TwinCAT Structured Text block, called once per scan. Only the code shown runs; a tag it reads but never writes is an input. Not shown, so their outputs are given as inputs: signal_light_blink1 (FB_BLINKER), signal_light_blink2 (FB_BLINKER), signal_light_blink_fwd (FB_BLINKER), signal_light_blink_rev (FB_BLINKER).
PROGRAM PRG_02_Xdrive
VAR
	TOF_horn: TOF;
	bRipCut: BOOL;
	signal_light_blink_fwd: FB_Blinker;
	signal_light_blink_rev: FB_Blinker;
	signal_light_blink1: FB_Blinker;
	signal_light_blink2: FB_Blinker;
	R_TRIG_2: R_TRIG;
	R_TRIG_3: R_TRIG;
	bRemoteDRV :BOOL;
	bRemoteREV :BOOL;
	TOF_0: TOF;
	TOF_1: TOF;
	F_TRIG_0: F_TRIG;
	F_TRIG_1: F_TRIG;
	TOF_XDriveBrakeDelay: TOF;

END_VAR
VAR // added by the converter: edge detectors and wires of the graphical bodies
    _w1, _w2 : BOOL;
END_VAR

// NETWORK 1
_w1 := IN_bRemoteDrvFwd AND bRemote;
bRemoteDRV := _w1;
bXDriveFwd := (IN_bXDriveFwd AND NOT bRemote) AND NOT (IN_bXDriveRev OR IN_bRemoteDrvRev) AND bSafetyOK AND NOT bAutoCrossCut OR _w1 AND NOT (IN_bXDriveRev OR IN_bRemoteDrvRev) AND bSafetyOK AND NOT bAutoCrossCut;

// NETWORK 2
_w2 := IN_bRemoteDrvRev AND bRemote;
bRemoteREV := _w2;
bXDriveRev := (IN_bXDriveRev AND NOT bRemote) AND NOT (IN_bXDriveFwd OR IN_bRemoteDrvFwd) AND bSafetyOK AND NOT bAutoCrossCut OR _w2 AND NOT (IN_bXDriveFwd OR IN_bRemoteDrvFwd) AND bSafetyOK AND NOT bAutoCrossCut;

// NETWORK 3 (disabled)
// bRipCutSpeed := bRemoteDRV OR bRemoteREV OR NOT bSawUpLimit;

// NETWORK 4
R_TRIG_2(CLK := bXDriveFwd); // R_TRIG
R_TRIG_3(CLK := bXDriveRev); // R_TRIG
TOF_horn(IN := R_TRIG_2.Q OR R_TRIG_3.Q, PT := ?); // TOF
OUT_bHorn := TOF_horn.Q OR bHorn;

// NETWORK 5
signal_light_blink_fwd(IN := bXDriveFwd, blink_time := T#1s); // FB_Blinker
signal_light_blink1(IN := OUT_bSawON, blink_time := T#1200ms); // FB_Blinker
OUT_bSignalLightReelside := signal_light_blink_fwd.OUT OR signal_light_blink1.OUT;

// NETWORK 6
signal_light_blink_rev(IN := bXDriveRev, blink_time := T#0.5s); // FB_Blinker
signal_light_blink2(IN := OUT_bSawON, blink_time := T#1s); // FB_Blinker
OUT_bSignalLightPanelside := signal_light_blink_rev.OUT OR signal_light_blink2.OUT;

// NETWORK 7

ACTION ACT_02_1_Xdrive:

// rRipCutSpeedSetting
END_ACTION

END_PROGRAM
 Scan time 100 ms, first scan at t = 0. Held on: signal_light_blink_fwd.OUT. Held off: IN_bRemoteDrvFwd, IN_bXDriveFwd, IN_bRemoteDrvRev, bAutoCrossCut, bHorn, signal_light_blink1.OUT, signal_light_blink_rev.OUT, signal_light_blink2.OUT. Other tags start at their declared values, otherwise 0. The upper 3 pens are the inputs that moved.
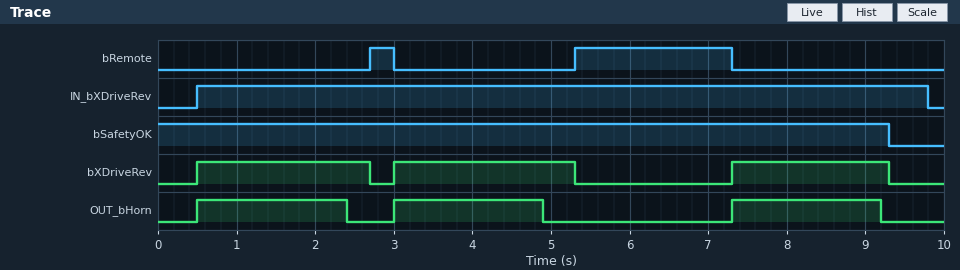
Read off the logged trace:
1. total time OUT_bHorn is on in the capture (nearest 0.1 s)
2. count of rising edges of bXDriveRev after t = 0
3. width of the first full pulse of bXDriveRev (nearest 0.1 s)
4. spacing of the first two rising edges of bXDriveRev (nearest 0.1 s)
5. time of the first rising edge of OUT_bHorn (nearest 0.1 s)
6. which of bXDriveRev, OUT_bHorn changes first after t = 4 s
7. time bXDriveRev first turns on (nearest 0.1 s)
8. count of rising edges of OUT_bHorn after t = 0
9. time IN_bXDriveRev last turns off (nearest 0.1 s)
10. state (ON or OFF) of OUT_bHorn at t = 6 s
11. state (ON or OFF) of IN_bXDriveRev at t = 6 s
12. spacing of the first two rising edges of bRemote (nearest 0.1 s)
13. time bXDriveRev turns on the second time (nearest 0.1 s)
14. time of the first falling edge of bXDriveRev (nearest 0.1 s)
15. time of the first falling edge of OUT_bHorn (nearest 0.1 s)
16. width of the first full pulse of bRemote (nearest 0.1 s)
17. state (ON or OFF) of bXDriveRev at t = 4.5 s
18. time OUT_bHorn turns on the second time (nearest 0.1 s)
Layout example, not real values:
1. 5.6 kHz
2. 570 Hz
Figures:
1. 5.7 s
2. 3
3. 2.2 s
4. 2.5 s
5. 0.5 s
6. OUT_bHorn
7. 0.5 s
8. 3
9. 9.8 s
10. OFF
11. ON
12. 2.6 s
13. 3.0 s
14. 2.7 s
15. 2.4 s
16. 0.3 s
17. ON
18. 3.0 s
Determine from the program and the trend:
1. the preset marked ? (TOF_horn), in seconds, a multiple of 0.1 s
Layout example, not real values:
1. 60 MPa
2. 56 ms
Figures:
1. 1.8 s
